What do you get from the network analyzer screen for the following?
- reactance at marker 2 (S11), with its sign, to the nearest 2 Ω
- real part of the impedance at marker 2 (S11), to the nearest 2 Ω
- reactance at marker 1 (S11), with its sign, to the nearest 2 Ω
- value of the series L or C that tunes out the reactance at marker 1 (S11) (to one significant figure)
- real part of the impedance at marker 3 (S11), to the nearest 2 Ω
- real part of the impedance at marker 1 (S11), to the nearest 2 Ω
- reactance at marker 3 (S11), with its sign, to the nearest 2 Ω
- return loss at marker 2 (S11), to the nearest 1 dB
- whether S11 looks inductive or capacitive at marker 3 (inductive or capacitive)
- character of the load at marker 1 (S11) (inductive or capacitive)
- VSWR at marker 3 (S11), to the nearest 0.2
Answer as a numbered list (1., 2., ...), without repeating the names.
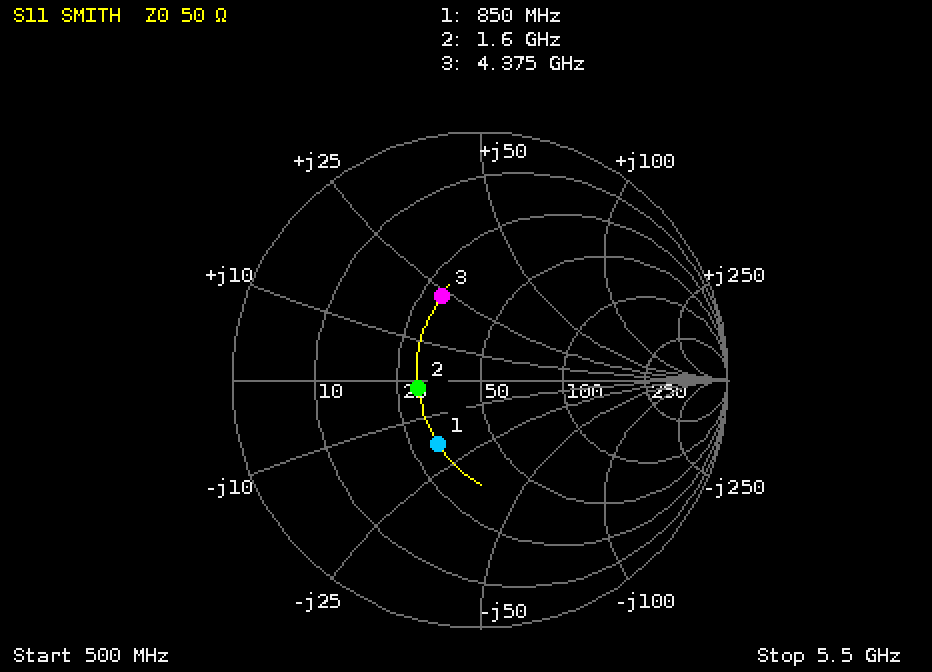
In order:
1. -2 Ω
2. 30 Ω
3. -18 Ω
4. 3 nH
5. 30 Ω
6. 32 Ω
7. +24 Ω
8. 12 dB
9. inductive
10. capacitive
11. 2.2
